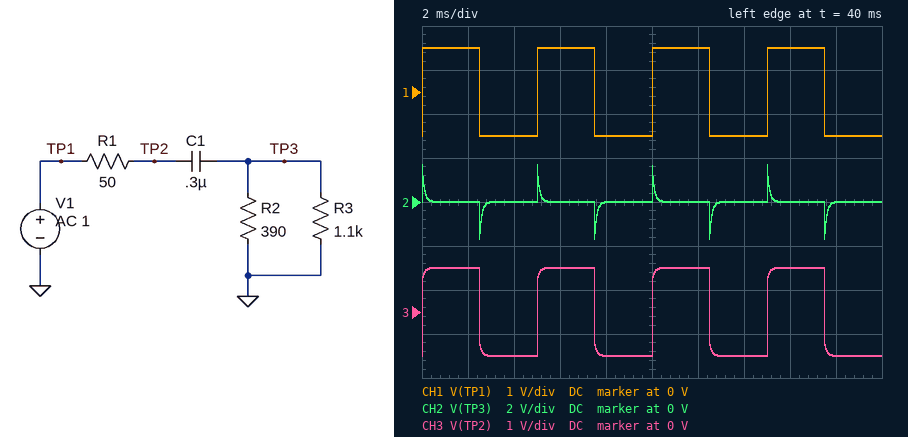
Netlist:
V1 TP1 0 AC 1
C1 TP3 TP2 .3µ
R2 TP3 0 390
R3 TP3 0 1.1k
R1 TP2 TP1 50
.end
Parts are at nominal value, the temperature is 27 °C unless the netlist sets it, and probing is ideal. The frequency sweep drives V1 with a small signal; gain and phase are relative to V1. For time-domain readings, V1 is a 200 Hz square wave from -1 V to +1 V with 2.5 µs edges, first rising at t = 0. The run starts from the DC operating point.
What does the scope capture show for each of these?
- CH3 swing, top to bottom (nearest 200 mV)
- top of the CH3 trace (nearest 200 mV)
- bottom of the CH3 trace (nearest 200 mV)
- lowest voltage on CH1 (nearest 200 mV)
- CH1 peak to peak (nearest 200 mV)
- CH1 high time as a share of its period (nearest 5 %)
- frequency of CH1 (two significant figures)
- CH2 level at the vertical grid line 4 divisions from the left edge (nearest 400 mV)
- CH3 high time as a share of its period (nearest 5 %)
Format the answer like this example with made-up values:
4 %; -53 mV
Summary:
2.0 V; 1.0 V; -1.0 V; -1.0 V; 2.0 V; 50 %; 200 Hz; 0 V; 50 %
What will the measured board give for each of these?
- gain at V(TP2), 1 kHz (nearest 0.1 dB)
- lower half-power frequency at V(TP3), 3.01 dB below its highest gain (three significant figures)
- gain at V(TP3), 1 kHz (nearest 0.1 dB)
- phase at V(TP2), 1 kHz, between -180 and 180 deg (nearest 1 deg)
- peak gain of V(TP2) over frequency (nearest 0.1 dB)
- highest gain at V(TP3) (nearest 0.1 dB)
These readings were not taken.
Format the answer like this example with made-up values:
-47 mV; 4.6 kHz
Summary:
-0.4 dB; 1.57 kHz; -6.8 dB; -4 deg; 0 dB; -1.4 dB
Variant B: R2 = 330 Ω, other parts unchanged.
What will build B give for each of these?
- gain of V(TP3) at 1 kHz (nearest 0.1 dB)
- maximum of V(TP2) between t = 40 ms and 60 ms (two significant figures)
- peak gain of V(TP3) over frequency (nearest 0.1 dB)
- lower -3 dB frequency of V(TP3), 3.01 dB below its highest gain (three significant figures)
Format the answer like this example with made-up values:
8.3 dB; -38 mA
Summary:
-7.6 dB; 1.0 V; -1.6 dB; 1.75 kHz
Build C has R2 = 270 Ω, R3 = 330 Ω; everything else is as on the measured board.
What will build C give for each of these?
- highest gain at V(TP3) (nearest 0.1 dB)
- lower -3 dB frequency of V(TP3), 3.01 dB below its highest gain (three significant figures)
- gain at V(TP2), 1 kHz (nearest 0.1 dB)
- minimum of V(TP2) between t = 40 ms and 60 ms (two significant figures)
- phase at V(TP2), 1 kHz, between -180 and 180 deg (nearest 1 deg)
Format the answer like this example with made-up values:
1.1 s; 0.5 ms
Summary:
-2.5 dB; 2.67 kHz; -0.2 dB; -1.0 V; -5 deg
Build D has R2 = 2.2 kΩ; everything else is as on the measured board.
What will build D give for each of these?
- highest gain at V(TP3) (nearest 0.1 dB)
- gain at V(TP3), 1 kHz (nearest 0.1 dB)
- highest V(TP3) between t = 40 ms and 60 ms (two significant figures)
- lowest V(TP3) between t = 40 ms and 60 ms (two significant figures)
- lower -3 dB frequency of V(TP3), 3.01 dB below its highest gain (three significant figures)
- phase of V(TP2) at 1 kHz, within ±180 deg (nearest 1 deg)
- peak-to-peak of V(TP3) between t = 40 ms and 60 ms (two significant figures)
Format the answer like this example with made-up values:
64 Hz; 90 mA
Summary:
-0.6 dB; -2.2 dB; 1.9 V; -1.9 V; 677 Hz; -2 deg; 3.7 V
